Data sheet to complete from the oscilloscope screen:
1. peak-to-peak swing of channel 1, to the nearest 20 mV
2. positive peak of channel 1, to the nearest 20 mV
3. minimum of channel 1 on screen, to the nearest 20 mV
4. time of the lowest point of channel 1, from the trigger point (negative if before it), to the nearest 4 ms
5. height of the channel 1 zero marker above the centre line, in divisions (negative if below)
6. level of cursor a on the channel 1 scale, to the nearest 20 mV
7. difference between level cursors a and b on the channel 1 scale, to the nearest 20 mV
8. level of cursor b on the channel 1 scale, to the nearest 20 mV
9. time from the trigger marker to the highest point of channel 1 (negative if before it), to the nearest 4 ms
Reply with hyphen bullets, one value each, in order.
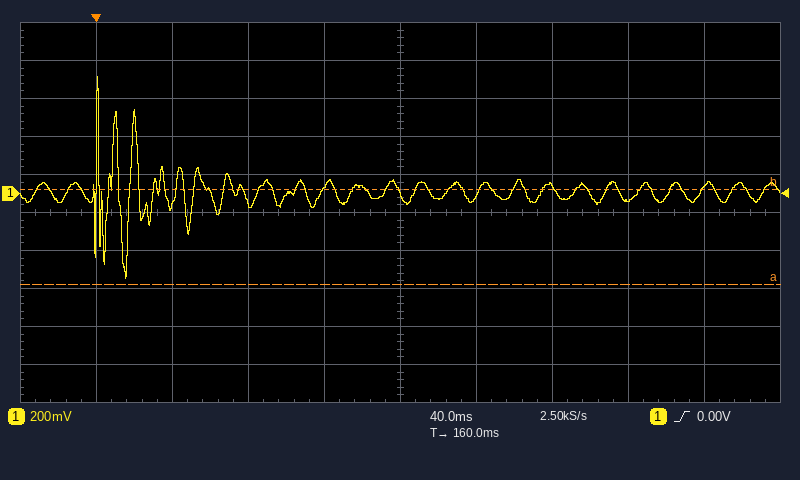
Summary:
- 1.06 V
- 620 mV
- -440 mV
- +16 ms
- +0.5 div
- -480 mV
- 500 mV
- 20 mV
- 0 ms
